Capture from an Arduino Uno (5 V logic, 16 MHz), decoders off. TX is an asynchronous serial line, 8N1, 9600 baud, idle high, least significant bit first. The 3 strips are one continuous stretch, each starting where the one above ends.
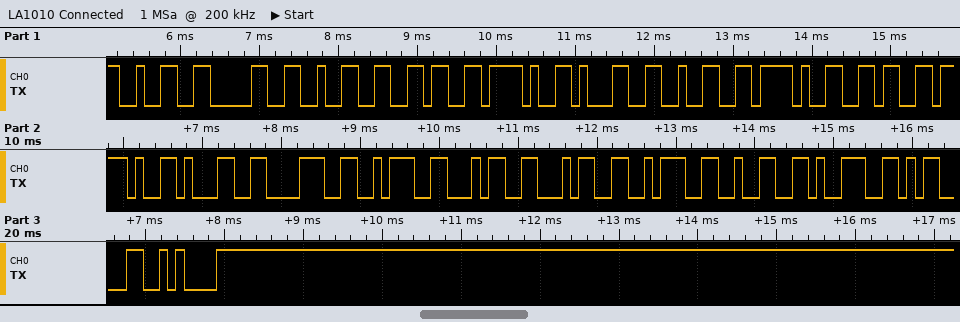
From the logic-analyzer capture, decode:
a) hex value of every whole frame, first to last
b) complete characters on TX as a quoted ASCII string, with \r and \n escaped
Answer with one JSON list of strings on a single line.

["32 30 32 36 2F 31 32 2F 36 2F 31 38 3A 34 34 3A 32 39 0D 0A", "\"2026/12/6/18:44:29\\r\\n\""]
